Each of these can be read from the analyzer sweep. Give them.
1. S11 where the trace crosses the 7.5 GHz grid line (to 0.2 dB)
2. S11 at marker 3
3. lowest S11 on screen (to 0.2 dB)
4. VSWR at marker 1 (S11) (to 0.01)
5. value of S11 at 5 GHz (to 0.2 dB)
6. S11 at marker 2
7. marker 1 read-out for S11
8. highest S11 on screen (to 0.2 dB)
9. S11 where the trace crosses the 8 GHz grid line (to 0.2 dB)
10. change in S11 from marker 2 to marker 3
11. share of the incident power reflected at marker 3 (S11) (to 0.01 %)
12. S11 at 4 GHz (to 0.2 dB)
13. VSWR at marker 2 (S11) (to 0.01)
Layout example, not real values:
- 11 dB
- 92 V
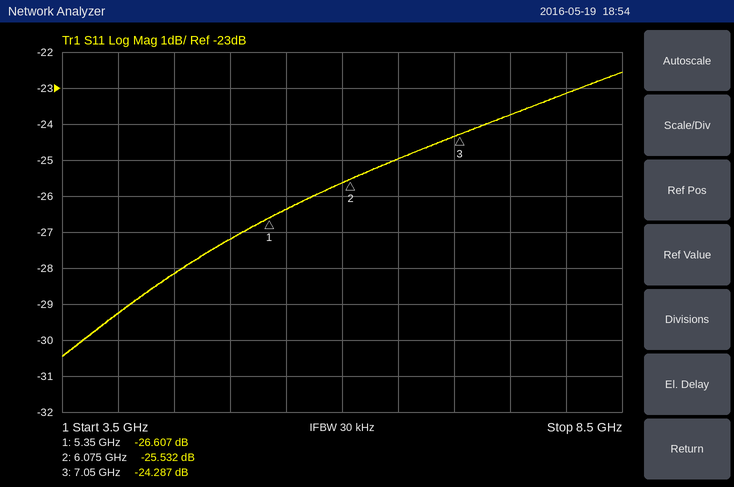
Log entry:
- -23.8 dB
- -24.287 dB
- -30.4 dB
- 1.10
- -27.2 dB
- -25.532 dB
- -26.607 dB
- -22.6 dB
- -23.2 dB
- 1.245 dB
- 0.37 %
- -29.2 dB
- 1.11
